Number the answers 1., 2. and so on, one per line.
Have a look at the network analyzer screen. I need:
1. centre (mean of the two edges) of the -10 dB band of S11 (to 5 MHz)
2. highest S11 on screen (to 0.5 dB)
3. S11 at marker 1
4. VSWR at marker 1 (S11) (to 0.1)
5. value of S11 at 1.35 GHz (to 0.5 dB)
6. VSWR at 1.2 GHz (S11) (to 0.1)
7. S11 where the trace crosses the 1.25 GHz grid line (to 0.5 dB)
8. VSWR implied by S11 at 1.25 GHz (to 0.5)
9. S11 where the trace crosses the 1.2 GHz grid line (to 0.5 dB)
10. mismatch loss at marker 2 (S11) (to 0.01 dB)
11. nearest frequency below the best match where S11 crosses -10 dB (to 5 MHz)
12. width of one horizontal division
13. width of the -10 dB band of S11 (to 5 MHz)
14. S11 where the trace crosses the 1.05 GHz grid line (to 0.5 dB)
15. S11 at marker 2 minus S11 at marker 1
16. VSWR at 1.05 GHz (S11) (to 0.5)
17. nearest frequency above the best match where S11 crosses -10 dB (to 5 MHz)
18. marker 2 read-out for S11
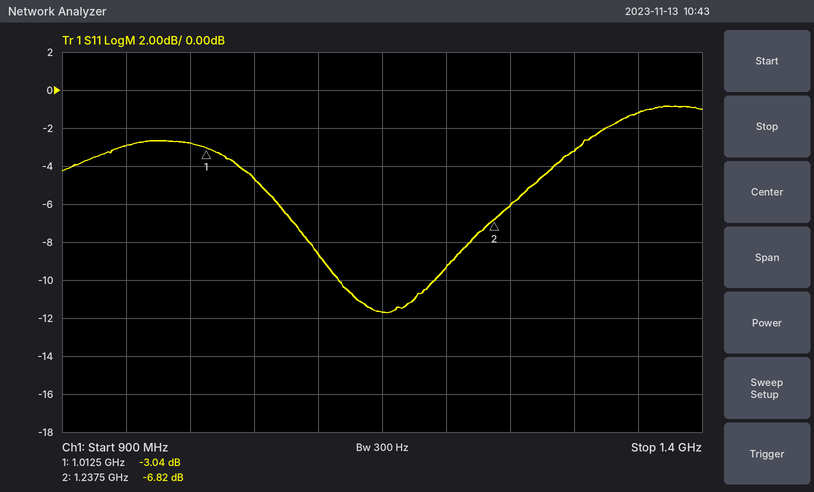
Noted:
1. 1.155 GHz
2. -1.0 dB
3. -3.04 dB
4. 5.8
5. -1.0 dB
6. 2.0
7. -6.0 dB
8. 3.0
9. -9.5 dB
10. 1.01 dB
11. 1.115 GHz
12. 50 MHz
13. 75 MHz
14. -4.5 dB
15. -3.78 dB
16. 4.0
17. 1.190 GHz
18. -6.82 dB
